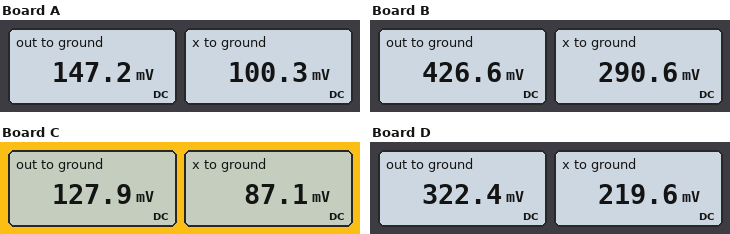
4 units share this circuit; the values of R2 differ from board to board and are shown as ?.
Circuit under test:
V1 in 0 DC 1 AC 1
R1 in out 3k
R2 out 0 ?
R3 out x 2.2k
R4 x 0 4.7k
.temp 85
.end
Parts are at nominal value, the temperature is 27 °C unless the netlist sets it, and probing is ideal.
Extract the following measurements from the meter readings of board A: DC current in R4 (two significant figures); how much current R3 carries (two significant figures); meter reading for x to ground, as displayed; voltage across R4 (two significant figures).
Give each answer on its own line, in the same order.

21 µA
21 µA
100.3 mV
100 mV
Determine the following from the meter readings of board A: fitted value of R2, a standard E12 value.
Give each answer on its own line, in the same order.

560 Ω
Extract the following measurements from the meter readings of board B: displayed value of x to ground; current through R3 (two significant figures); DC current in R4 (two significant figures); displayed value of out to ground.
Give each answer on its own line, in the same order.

290.6 mV
62 µA
62 µA
426.6 mV
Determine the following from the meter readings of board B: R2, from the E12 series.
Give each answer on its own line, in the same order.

3.3 kΩ
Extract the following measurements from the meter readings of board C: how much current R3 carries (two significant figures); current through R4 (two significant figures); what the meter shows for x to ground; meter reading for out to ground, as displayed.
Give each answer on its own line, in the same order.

19 µA
19 µA
87.1 mV
127.9 mV
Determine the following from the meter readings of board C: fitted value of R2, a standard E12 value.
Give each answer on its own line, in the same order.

470 Ω
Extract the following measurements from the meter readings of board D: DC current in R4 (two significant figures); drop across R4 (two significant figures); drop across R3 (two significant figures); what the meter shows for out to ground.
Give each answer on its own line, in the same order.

47 µA
220 mV
100 mV
322.4 mV
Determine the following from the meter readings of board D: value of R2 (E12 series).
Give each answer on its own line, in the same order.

1.8 kΩ
